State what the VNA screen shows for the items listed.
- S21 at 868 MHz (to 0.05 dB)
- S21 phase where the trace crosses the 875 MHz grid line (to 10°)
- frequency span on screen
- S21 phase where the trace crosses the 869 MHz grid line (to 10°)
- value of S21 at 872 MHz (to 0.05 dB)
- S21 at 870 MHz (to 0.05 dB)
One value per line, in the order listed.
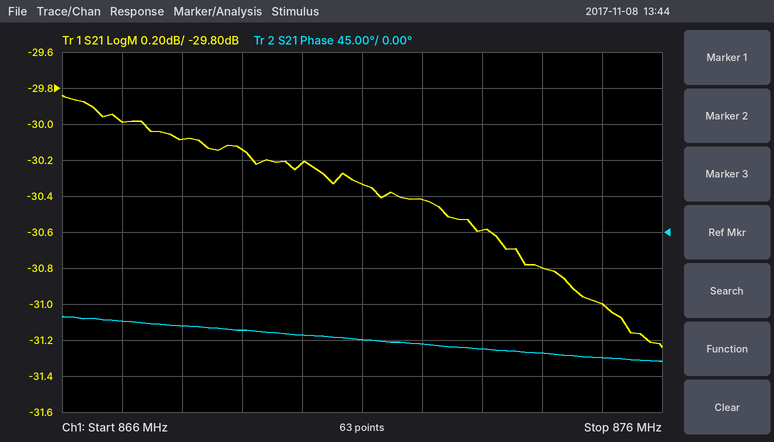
-30.10 dB
-160°
10 MHz
-120°
-30.40 dB
-30.20 dB
